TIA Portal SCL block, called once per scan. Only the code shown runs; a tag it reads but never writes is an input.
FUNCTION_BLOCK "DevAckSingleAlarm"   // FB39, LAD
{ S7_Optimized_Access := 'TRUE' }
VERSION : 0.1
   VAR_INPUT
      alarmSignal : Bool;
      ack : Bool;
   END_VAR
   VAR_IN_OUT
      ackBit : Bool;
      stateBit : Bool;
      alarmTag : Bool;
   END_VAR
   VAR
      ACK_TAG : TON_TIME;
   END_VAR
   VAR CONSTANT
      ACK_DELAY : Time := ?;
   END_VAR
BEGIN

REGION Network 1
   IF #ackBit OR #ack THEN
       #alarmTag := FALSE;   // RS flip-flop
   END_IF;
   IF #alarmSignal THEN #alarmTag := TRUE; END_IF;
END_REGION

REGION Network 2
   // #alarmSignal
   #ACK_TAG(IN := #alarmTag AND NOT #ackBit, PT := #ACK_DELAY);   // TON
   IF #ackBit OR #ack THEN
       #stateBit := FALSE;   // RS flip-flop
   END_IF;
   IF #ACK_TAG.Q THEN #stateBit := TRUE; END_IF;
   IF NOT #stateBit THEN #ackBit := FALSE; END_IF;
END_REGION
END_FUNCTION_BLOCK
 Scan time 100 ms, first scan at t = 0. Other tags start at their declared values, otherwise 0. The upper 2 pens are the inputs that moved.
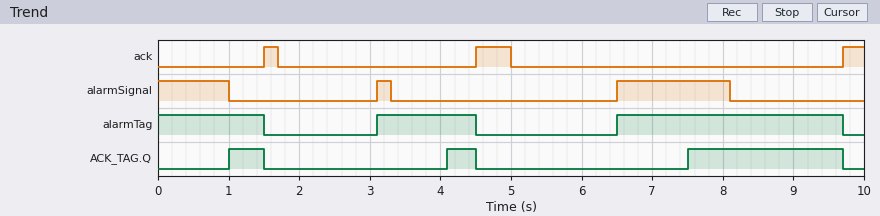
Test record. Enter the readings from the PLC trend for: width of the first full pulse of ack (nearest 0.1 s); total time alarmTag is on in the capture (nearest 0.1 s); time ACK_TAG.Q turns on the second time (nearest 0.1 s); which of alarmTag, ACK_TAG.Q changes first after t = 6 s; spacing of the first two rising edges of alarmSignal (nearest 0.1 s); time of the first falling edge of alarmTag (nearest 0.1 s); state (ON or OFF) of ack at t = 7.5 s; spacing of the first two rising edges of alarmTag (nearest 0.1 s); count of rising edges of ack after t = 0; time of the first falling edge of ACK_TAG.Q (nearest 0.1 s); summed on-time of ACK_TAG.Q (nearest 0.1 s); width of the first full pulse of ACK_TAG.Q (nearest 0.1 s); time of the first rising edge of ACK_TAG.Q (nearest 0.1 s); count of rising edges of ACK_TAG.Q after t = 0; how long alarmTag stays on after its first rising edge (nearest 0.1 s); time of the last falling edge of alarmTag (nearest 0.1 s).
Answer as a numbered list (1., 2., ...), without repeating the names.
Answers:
1. 0.2 s
2. 6.1 s
3. 4.1 s
4. alarmTag
5. 3.4 s
6. 1.5 s
7. OFF
8. 3.4 s
9. 3
10. 1.5 s
11. 3.1 s
12. 0.5 s
13. 1.0 s
14. 3
15. 1.4 s
16. 9.7 s
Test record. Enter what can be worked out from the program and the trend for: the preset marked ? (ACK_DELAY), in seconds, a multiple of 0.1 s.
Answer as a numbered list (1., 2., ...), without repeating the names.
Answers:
1. 1.0 s
